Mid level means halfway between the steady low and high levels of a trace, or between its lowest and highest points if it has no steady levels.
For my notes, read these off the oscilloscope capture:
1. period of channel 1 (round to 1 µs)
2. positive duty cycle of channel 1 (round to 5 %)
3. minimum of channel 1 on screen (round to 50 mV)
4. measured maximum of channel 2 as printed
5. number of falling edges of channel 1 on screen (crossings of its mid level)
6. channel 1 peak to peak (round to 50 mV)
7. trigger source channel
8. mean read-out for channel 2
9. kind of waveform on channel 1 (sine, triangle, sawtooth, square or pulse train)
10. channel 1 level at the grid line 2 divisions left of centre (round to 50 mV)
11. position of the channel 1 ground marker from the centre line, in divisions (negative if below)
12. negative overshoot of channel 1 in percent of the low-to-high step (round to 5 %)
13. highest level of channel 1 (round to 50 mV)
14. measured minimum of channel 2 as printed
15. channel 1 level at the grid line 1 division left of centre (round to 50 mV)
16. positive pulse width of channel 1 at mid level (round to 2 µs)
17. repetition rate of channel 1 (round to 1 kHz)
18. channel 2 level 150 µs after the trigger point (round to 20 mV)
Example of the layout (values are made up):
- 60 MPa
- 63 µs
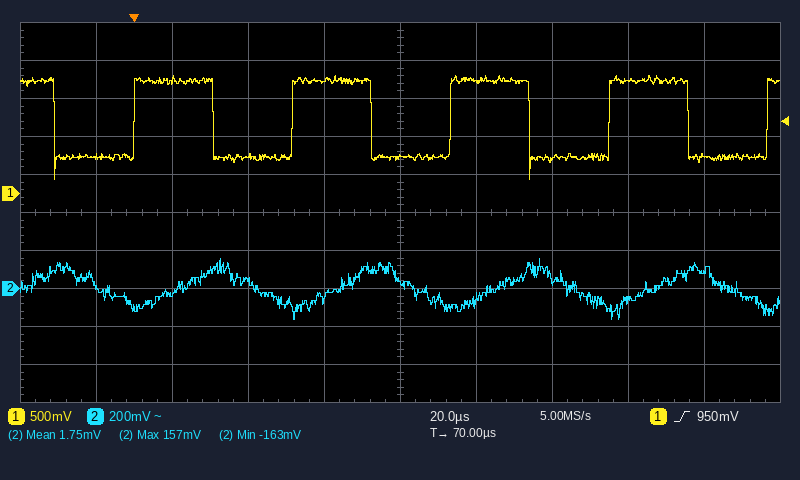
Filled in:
- 42 µs
- 50 %
- 200 mV
- 157 mV
- 5
- 1.35 V
- channel 1
- 1.75 mV
- square
- 500 mV
- +0.5 div
- 30 %
- 1.55 V
- -163 mV
- 1.50 V
- 20 µs
- 24 kHz
- 100 mV
